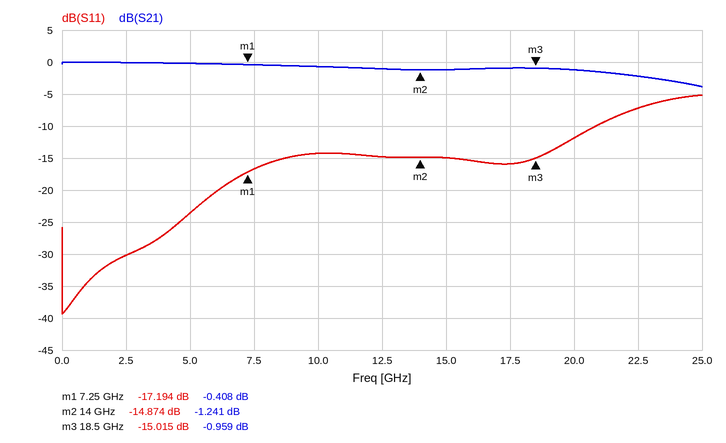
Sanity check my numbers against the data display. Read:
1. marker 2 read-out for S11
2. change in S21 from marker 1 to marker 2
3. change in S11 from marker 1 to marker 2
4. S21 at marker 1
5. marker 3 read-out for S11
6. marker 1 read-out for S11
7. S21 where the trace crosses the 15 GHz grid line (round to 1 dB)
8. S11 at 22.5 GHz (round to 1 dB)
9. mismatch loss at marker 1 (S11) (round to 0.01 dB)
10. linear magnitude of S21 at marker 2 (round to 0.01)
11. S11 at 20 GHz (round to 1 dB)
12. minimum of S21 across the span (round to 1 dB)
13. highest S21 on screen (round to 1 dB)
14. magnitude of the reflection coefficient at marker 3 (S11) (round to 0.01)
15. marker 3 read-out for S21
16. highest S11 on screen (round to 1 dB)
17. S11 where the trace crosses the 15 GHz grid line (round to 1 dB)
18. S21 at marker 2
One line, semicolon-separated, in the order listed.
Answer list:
-14.874 dB; -0.833 dB; 2.320 dB; -0.408 dB; -15.015 dB; -17.194 dB; -1 dB; -7 dB; 0.08 dB; 0.87; -12 dB; -4 dB; 0 dB; 0.18; -0.959 dB; -5 dB; -15 dB; -1.241 dB
